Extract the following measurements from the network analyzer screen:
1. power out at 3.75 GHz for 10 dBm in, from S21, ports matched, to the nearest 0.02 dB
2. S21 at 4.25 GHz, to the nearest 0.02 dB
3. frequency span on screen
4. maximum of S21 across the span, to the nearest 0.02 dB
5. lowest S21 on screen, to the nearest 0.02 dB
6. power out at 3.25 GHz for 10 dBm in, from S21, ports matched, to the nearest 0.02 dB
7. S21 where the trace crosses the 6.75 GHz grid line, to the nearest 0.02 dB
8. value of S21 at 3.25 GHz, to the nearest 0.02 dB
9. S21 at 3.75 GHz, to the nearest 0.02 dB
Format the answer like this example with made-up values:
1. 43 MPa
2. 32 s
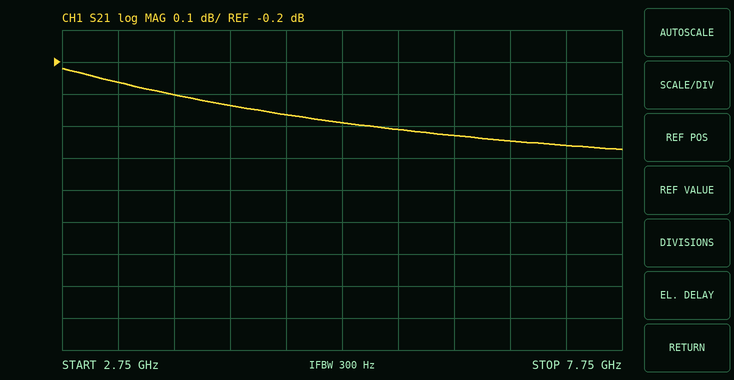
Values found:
1. 9.70 dBm
2. -0.34 dB
3. 5 GHz
4. -0.22 dB
5. -0.48 dB
6. 9.74 dBm
7. -0.44 dB
8. -0.26 dB
9. -0.30 dB
